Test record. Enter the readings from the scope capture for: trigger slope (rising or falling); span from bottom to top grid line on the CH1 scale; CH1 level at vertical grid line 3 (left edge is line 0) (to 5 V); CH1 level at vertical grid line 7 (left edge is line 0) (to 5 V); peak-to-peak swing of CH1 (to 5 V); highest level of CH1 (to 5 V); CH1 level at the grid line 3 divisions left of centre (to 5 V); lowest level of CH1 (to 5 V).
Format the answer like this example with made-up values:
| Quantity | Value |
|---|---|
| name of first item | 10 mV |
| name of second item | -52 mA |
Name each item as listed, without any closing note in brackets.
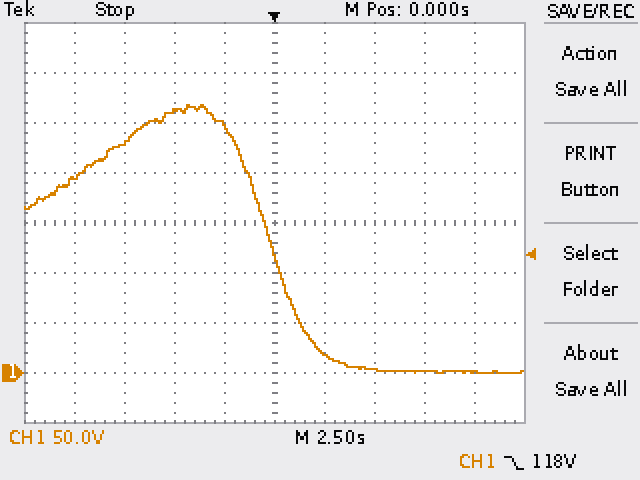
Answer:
| Quantity | Value |
|---|---|
| trigger slope | falling |
| span from bottom to top grid line on the CH1 scale | 400 V |
| CH1 level at vertical grid line 3 (left edge is line 0) | 260 V |
| CH1 level at vertical grid line 7 (left edge is line 0) | 5 V |
| peak-to-peak swing of CH1 | 270 V |
| highest level of CH1 | 270 V |
| CH1 level at the grid line 3 divisions left of centre | 230 V |
| lowest level of CH1 | 0 V |
